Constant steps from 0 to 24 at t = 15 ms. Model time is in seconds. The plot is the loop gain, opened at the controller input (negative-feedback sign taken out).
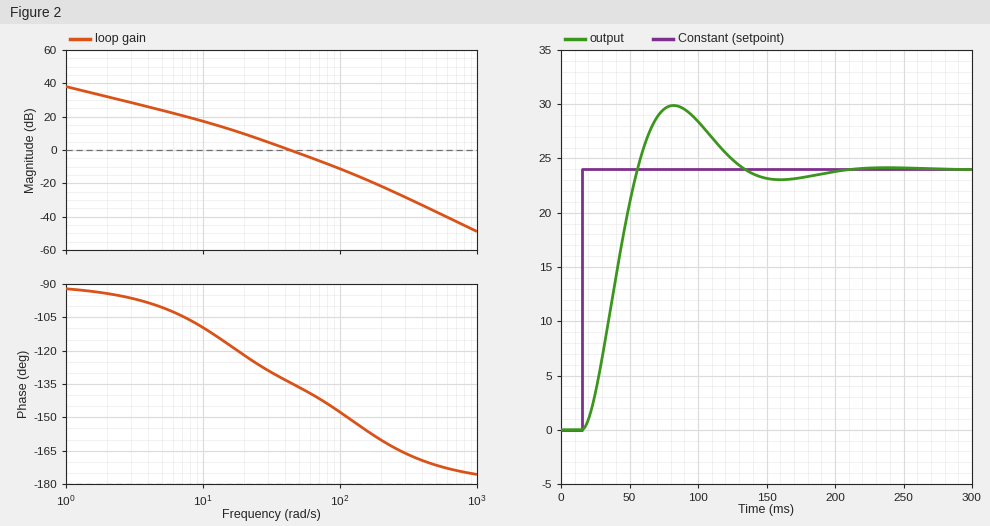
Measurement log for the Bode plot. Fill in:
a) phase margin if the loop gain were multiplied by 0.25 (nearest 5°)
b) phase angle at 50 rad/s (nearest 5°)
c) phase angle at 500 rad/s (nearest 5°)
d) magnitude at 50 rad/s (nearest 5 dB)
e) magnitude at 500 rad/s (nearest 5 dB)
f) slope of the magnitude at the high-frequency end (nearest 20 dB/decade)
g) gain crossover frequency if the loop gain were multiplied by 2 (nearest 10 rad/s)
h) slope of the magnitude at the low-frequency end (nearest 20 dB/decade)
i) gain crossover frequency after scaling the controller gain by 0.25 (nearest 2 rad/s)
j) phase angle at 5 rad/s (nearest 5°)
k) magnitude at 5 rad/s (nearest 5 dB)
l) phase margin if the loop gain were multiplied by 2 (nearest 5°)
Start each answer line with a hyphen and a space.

- 60°
- -135°
- -170°
- 0 dB
- -35 dB
- -40 dB/decade
- 70 rad/s
- -20 dB/decade
- 16 rad/s
- -100°
- 25 dB
- 40°
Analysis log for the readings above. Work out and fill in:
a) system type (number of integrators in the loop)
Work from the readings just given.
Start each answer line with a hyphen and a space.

- 1
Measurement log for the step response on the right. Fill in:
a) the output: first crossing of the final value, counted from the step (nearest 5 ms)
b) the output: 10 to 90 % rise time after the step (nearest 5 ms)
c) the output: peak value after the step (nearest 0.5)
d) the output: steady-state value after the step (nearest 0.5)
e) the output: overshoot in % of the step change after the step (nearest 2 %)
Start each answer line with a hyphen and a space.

- 40 ms
- 30 ms
- 30.0
- 24.0
- 24 %
